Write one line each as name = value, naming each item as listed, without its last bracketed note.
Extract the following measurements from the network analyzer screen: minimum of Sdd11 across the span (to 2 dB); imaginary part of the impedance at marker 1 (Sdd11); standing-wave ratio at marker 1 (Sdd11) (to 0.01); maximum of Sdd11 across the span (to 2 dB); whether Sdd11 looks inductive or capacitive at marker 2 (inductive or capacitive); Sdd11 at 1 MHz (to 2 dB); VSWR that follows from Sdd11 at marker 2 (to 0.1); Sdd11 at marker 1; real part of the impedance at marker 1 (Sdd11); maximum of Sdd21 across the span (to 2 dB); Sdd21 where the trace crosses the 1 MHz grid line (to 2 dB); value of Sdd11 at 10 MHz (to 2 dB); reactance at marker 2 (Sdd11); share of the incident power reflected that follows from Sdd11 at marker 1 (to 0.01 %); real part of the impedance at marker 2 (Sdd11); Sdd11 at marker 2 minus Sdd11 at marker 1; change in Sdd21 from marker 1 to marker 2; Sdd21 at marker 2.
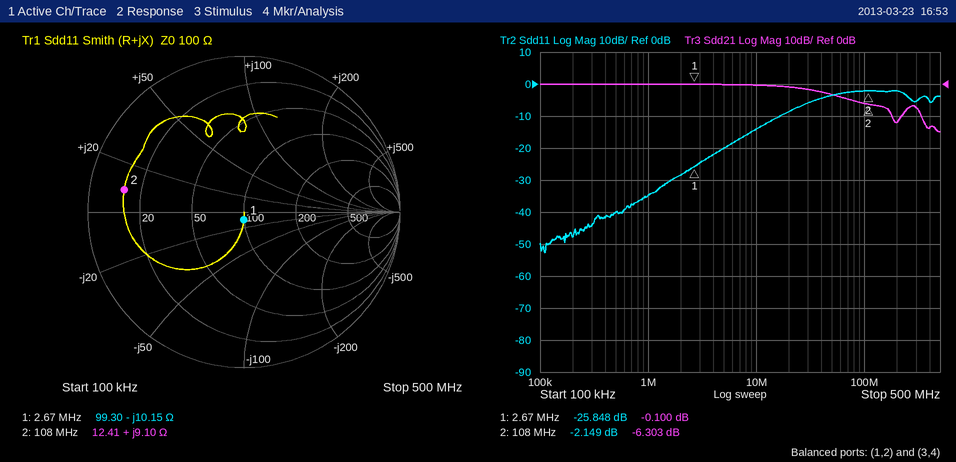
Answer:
minimum of Sdd11 across the span = -52 dB
imaginary part of the impedance at marker 1 = -10.15 Ω
standing-wave ratio at marker 1 (Sdd11) = 1.11
maximum of Sdd11 across the span = -2 dB
whether Sdd11 looks inductive or capacitive at marker 2 = inductive
Sdd11 at 1 MHz = -34 dB
VSWR that follows from Sdd11 at marker 2 = 8.1
Sdd11 at marker 1 = -25.848 dB
real part of the impedance at marker 1 = 99.30 Ω
maximum of Sdd21 across the span = 0 dB
Sdd21 where the trace crosses the 1 MHz grid line = 0 dB
value of Sdd11 at 10 MHz = -14 dB
reactance at marker 2 = +9.10 Ω
share of the incident power reflected that follows from Sdd11 at marker 1 = 0.26 %
real part of the impedance at marker 2 = 12.41 Ω
Sdd11 at marker 2 minus Sdd11 at marker 1 = 23.699 dB
change in Sdd21 from marker 1 to marker 2 = -6.203 dB
Sdd21 at marker 2 = -6.303 dB
